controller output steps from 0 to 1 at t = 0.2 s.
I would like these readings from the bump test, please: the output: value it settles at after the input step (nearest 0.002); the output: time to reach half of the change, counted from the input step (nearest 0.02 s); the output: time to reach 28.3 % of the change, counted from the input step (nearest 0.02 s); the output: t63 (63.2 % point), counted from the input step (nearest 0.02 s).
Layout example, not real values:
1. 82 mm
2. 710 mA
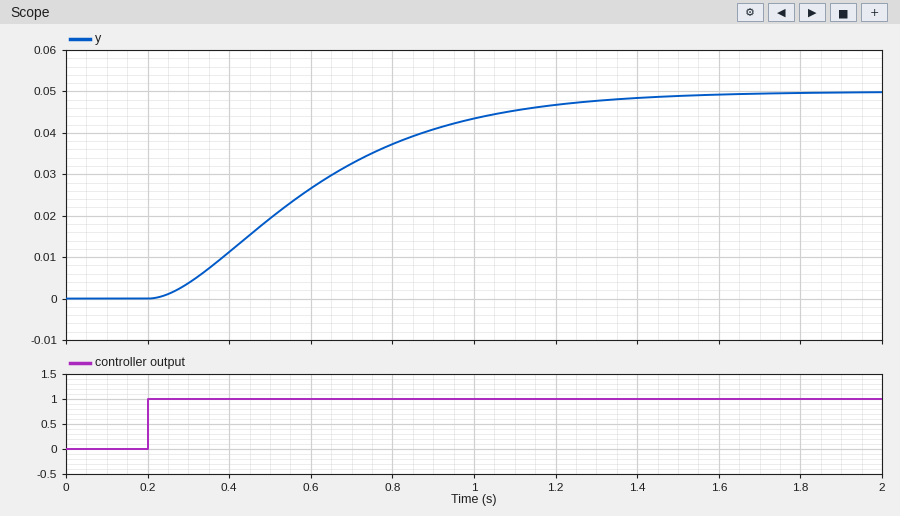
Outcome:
1. 0.050
2. 0.38 s
3. 0.24 s
4. 0.48 s
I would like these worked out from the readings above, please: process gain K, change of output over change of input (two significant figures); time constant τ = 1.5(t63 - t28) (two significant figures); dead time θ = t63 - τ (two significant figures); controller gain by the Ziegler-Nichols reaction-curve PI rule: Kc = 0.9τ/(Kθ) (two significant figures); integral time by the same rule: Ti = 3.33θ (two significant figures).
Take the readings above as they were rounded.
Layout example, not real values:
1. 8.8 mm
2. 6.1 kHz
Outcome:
1. 0.050
2. 0.36 s
3. 0.12 s
4. 54
5. 0.40 s
